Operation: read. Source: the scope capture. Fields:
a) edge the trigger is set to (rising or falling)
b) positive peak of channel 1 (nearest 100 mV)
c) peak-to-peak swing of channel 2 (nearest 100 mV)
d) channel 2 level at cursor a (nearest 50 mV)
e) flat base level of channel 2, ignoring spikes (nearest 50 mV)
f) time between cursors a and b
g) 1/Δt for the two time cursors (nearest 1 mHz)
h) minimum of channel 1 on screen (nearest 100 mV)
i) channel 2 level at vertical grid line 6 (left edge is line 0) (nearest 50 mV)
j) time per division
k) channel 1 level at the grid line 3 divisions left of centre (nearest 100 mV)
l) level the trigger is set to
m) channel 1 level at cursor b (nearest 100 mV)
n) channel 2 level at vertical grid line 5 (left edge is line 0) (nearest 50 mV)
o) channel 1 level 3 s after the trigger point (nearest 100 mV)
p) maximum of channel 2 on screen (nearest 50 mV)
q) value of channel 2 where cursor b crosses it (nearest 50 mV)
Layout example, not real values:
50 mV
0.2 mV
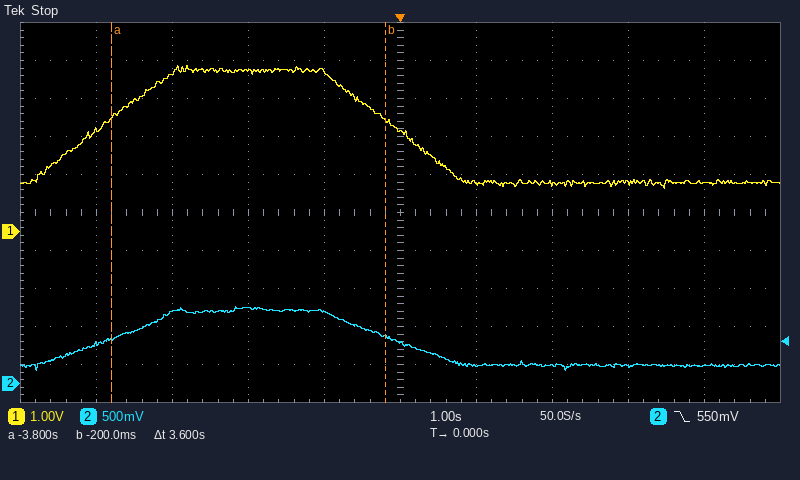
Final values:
falling
4.4 V
800 mV
600 mV
250 mV
3.6 s
278 mHz
1.1 V
250 mV
1 s
4.2 V
550 mV
2.9 V
550 mV
1.3 V
1.00 V
600 mV
